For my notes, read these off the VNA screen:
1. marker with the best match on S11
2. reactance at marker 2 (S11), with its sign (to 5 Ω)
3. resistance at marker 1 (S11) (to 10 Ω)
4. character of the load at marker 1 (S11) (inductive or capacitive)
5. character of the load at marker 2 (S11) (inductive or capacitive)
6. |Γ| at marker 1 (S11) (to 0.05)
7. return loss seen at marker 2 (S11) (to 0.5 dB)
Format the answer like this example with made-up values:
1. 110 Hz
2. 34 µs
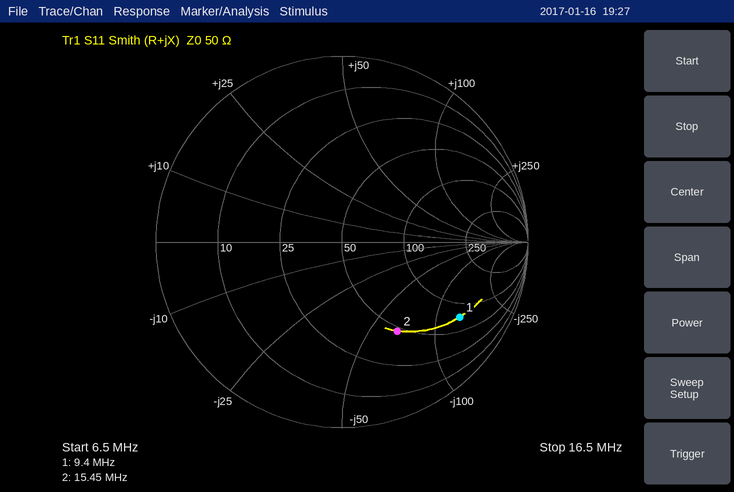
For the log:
1. marker 2
2. -65 Ω
3. 70 Ω
4. capacitive
5. capacitive
6. 0.75
7. 5.0 dB
